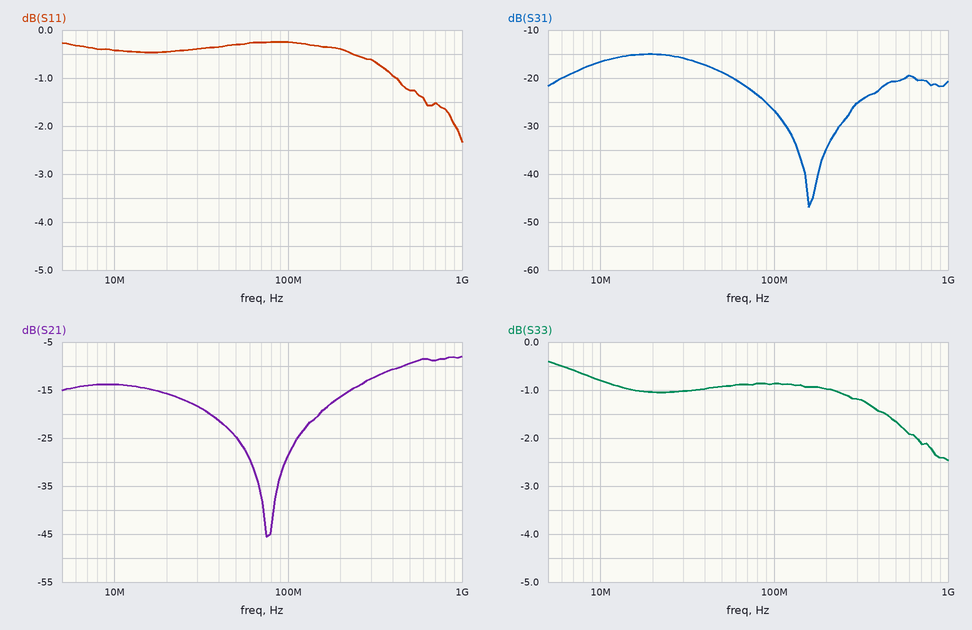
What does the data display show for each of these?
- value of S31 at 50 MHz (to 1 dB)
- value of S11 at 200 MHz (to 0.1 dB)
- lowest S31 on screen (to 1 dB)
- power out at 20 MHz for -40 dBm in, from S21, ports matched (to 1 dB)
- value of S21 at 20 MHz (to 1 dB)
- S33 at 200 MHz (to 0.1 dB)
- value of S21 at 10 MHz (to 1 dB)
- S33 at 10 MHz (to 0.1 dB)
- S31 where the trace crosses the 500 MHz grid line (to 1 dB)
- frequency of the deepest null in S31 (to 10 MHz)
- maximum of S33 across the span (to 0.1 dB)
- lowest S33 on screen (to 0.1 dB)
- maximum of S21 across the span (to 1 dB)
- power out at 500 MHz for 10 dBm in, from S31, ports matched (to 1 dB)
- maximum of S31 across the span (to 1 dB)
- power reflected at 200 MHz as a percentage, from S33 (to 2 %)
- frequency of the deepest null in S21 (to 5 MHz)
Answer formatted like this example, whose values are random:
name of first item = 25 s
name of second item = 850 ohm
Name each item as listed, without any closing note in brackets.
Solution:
value of S31 at 50 MHz = -19 dB
value of S11 at 200 MHz = -0.4 dB
lowest S31 on screen = -47 dB
power out at 20 MHz for -40 dBm in, from S21, ports matched = -56 dBm
value of S21 at 20 MHz = -16 dB
S33 at 200 MHz = -1.0 dB
value of S21 at 10 MHz = -14 dB
S33 at 10 MHz = -0.8 dB
S31 where the trace crosses the 500 MHz grid line = -21 dB
frequency of the deepest null in S31 = 160 MHz
maximum of S33 across the span = -0.4 dB
lowest S33 on screen = -2.5 dB
maximum of S21 across the span = -8 dB
power out at 500 MHz for 10 dBm in, from S31, ports matched = -11 dBm
maximum of S31 across the span = -15 dB
power reflected at 200 MHz as a percentage, from S33 = 80 %
frequency of the deepest null in S21 = 75 MHz
